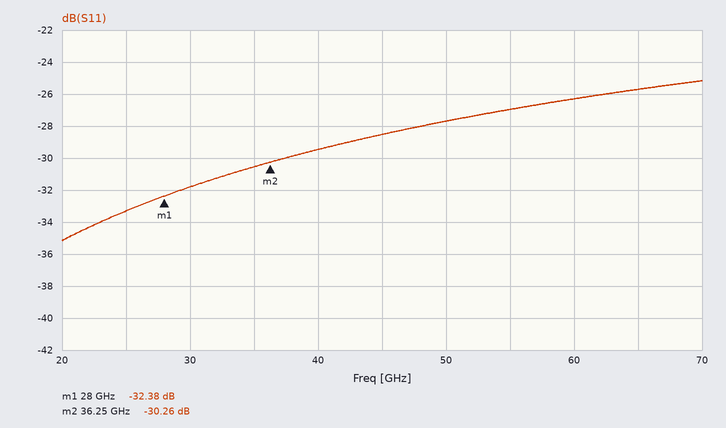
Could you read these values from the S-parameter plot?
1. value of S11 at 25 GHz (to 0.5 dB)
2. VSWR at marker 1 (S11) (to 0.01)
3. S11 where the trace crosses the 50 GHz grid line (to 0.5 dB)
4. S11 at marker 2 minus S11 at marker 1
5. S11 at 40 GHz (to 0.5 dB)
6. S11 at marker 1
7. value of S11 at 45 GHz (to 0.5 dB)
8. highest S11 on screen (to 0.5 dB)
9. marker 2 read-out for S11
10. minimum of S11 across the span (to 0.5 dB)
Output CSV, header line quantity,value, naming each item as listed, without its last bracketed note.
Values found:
quantity,value
value of S11 at 25 GHz,-33.5 dB
VSWR at marker 1 (S11),1.05
S11 where the trace crosses the 50 GHz grid line,-27.5 dB
S11 at marker 2 minus S11 at marker 1,2.12 dB
S11 at 40 GHz,-29.5 dB
S11 at marker 1,-32.38 dB
value of S11 at 45 GHz,-28.5 dB
highest S11 on screen,-25.0 dB
marker 2 read-out for S11,-30.26 dB
minimum of S11 across the span,-35.0 dB
